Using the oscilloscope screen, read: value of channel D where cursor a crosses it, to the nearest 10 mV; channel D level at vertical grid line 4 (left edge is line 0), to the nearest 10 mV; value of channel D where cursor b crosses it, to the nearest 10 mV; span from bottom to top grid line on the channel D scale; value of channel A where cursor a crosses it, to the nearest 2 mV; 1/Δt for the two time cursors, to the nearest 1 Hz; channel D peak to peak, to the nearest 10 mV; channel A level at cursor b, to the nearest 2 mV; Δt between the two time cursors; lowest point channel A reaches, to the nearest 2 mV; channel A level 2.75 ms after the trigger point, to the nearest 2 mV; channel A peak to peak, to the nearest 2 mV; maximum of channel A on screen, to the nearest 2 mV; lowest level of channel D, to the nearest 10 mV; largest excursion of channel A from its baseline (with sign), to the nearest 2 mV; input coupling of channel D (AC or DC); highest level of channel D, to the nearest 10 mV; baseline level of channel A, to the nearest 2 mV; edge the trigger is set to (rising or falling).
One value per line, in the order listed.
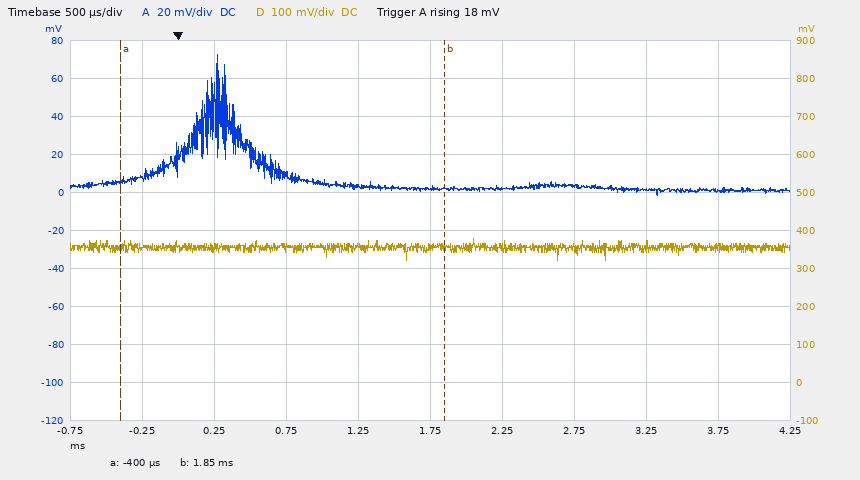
360 mV
360 mV
360 mV
1 V
6 mV
444 Hz
60 mV
2 mV
2.25 ms
-2 mV
4 mV
74 mV
72 mV
320 mV
+70 mV
DC
380 mV
2 mV
rising
